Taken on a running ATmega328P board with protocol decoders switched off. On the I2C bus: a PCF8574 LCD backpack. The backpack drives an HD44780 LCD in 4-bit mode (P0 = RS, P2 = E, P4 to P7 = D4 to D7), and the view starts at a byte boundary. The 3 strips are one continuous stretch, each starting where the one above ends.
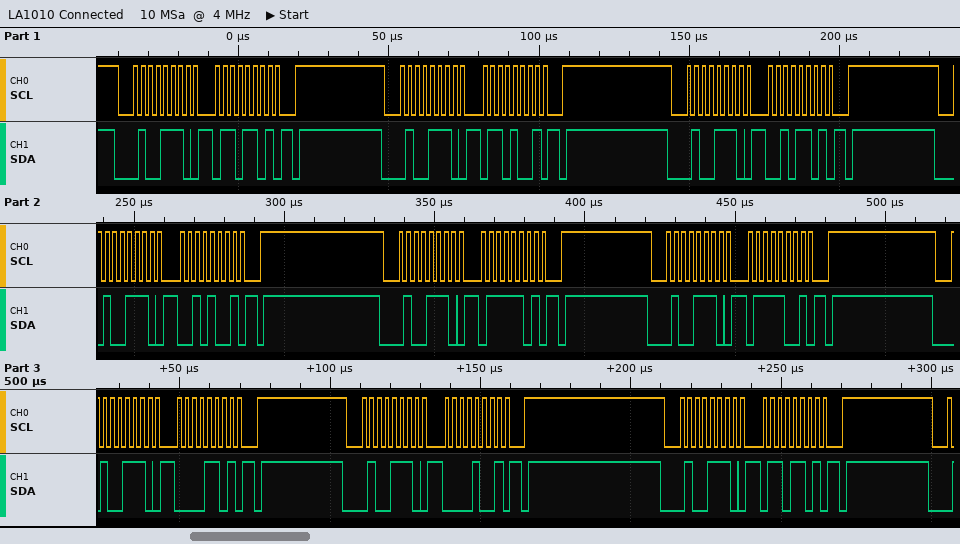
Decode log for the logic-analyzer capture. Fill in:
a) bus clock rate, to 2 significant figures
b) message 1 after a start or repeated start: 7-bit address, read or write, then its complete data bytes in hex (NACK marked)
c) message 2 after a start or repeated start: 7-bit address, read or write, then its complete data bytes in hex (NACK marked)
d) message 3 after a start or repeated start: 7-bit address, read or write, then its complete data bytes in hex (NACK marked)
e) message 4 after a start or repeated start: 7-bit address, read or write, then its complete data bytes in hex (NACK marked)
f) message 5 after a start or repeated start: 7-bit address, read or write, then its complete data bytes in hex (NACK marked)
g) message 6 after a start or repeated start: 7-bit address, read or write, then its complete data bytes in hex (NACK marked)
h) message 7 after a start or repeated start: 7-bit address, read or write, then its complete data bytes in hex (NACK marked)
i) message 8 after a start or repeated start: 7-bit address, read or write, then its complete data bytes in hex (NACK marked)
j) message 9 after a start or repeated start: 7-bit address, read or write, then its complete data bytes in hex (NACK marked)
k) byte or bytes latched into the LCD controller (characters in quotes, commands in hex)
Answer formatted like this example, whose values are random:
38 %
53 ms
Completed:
400 kHz
0x27 write: 6D
0x27 write: 69
0x27 write: 2D
0x27 write: 29
0x27 write: 7D
0x27 write: 79
0x27 write: 0D
0x27 write: 09
0x27 write: 6D
'b' 'p'
